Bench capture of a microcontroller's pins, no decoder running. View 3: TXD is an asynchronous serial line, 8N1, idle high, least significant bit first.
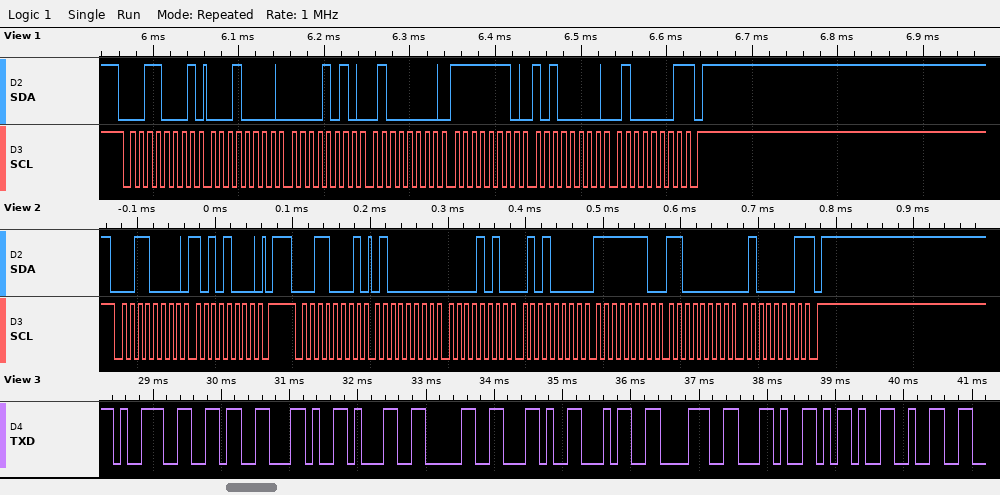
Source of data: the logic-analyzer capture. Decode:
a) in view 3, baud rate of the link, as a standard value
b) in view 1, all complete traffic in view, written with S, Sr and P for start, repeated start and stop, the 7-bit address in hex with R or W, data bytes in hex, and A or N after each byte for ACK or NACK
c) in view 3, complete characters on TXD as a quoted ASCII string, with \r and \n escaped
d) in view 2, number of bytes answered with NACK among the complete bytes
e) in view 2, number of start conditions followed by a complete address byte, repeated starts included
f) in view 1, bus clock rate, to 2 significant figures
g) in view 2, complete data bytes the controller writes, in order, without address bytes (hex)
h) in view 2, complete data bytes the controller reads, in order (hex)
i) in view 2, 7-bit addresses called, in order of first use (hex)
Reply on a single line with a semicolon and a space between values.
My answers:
9600 baud; S 18R A 10 A 0A A 40 A FE A A0 A 41 N P; "96,10,48,-2"; 1; 2; 100 kHz; A8; 40 0A 50 FE C0 41; 0x18
